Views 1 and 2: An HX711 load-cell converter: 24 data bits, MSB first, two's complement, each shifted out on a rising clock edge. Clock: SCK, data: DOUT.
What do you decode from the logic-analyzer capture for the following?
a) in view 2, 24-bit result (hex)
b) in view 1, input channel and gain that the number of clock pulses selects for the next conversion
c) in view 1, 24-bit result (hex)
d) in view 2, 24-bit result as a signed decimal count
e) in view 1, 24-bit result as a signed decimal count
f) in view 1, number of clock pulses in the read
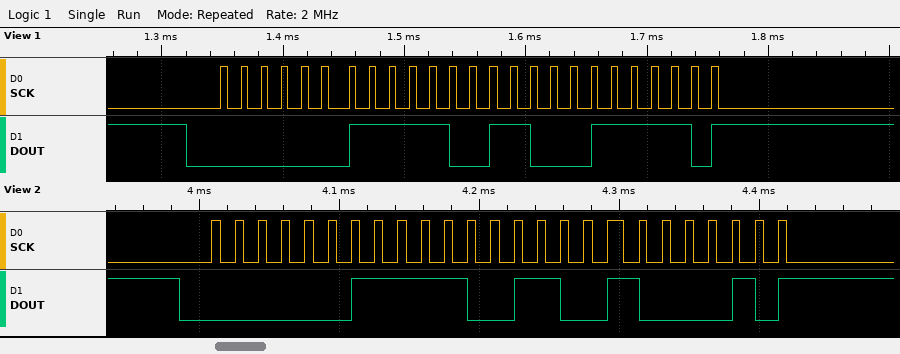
0x03E642
channel A, gain 128
0x03E63E
255554
255550
25
